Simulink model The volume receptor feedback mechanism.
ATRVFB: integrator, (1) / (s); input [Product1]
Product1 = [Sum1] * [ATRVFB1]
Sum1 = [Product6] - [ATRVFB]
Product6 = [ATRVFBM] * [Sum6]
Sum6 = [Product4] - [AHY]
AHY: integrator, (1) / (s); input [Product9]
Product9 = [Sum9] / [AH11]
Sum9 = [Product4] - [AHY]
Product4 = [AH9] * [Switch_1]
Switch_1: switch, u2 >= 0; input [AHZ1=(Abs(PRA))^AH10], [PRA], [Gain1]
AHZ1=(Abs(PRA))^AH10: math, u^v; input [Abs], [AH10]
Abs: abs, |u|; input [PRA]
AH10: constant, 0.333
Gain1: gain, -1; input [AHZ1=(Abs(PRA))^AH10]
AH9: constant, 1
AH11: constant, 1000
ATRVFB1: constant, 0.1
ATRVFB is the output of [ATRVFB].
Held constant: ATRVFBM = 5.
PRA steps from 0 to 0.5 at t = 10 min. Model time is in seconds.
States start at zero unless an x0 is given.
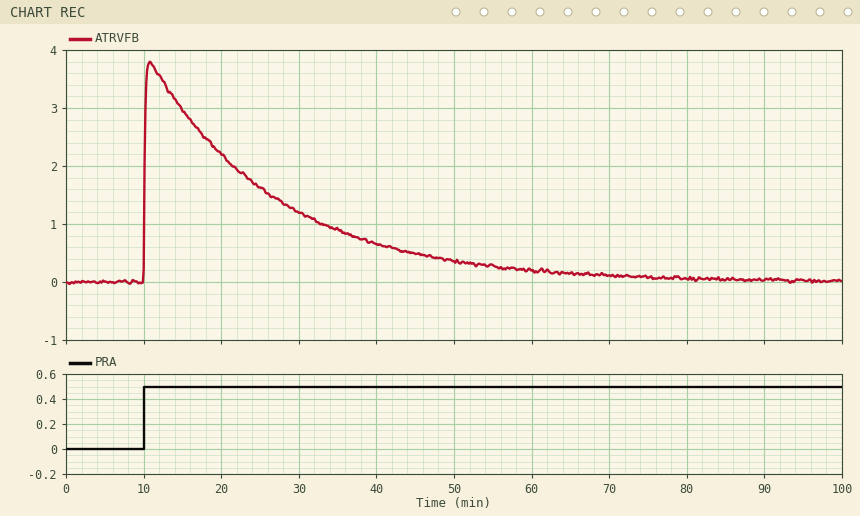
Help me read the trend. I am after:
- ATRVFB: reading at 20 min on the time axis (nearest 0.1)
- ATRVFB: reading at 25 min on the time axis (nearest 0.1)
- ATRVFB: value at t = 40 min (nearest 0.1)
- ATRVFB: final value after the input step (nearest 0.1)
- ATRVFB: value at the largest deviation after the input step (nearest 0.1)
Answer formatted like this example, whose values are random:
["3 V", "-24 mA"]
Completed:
["2.2", "1.6", "0.7", "0.0", "3.8"]
